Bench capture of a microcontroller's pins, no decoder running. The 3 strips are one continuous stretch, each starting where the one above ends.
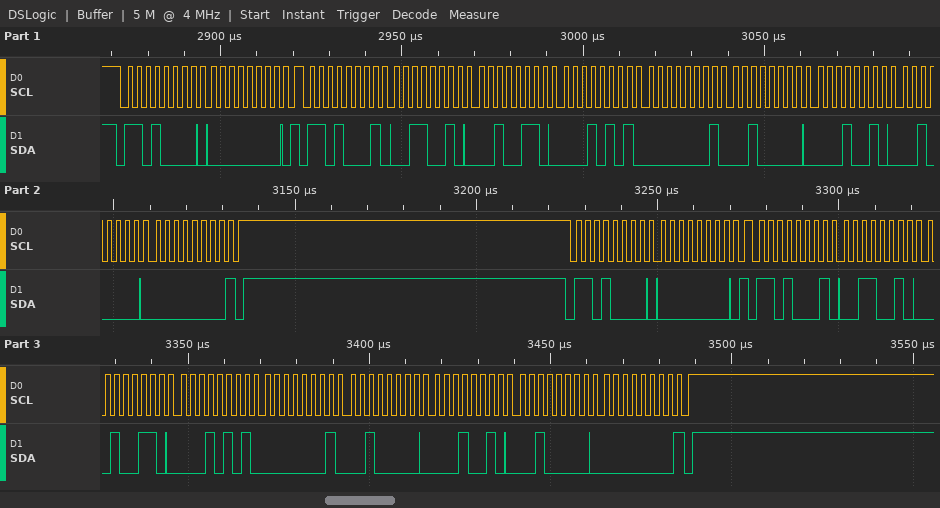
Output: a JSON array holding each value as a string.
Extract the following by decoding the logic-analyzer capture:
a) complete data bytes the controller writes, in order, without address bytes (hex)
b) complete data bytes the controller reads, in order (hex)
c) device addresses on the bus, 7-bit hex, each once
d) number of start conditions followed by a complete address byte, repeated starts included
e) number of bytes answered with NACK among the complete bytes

["00 00", "32 26 15 01 20 12 20 00 32 26 15 01 20 12 20 00", "0x68", "4", "2"]
